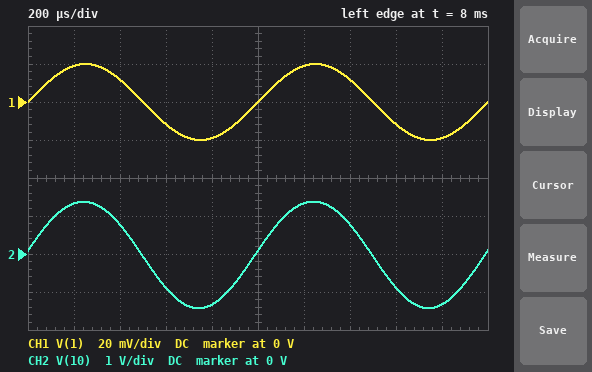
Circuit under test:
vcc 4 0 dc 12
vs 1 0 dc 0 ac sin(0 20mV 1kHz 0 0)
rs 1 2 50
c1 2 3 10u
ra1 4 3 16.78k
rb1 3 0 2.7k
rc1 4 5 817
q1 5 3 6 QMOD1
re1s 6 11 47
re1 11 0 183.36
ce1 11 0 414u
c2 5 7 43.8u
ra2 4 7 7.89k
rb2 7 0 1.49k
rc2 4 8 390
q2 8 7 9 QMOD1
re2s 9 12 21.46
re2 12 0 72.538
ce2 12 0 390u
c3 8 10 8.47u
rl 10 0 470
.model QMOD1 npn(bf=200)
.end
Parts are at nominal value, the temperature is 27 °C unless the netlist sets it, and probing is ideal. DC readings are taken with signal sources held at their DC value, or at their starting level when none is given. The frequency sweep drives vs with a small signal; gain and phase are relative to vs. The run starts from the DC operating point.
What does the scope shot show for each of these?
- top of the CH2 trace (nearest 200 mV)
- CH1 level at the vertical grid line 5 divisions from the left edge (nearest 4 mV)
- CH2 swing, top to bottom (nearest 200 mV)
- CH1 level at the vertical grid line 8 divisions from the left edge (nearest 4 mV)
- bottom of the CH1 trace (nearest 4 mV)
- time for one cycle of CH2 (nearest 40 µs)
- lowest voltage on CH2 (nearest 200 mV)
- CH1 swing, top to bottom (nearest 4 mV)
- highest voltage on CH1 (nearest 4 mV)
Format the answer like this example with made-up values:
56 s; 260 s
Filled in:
1.4 V; 0 V; 2.8 V; -12 mV; -20 mV; 1.00 ms; -1.4 V; 40 mV; 20 mV
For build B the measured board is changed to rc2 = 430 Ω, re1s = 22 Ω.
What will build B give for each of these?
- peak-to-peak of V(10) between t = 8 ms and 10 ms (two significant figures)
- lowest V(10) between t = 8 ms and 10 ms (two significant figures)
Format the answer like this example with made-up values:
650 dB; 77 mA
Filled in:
5.2 V; -2.8 V
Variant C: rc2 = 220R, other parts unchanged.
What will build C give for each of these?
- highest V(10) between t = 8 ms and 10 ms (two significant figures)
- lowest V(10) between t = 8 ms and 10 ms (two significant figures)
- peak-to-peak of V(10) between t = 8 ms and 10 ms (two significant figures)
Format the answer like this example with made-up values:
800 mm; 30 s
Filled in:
970 mV; -1.0 V; 2.0 V
